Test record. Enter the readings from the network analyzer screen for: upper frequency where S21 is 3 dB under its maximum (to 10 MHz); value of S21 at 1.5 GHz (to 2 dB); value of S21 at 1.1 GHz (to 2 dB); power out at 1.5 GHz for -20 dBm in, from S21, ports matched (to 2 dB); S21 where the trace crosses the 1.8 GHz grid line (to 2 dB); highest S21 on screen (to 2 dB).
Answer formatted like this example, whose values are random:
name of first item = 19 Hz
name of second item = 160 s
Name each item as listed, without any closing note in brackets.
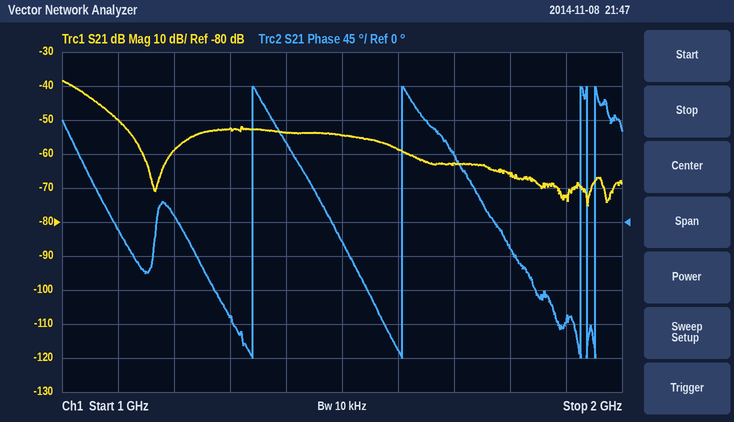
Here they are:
upper frequency where S21 is 3 dB under its maximum = 1.03 GHz
value of S21 at 1.5 GHz = -54 dB
value of S21 at 1.1 GHz = -50 dB
power out at 1.5 GHz for -20 dBm in, from S21, ports matched = -74 dBm
S21 where the trace crosses the 1.8 GHz grid line = -66 dB
highest S21 on screen = -38 dB
